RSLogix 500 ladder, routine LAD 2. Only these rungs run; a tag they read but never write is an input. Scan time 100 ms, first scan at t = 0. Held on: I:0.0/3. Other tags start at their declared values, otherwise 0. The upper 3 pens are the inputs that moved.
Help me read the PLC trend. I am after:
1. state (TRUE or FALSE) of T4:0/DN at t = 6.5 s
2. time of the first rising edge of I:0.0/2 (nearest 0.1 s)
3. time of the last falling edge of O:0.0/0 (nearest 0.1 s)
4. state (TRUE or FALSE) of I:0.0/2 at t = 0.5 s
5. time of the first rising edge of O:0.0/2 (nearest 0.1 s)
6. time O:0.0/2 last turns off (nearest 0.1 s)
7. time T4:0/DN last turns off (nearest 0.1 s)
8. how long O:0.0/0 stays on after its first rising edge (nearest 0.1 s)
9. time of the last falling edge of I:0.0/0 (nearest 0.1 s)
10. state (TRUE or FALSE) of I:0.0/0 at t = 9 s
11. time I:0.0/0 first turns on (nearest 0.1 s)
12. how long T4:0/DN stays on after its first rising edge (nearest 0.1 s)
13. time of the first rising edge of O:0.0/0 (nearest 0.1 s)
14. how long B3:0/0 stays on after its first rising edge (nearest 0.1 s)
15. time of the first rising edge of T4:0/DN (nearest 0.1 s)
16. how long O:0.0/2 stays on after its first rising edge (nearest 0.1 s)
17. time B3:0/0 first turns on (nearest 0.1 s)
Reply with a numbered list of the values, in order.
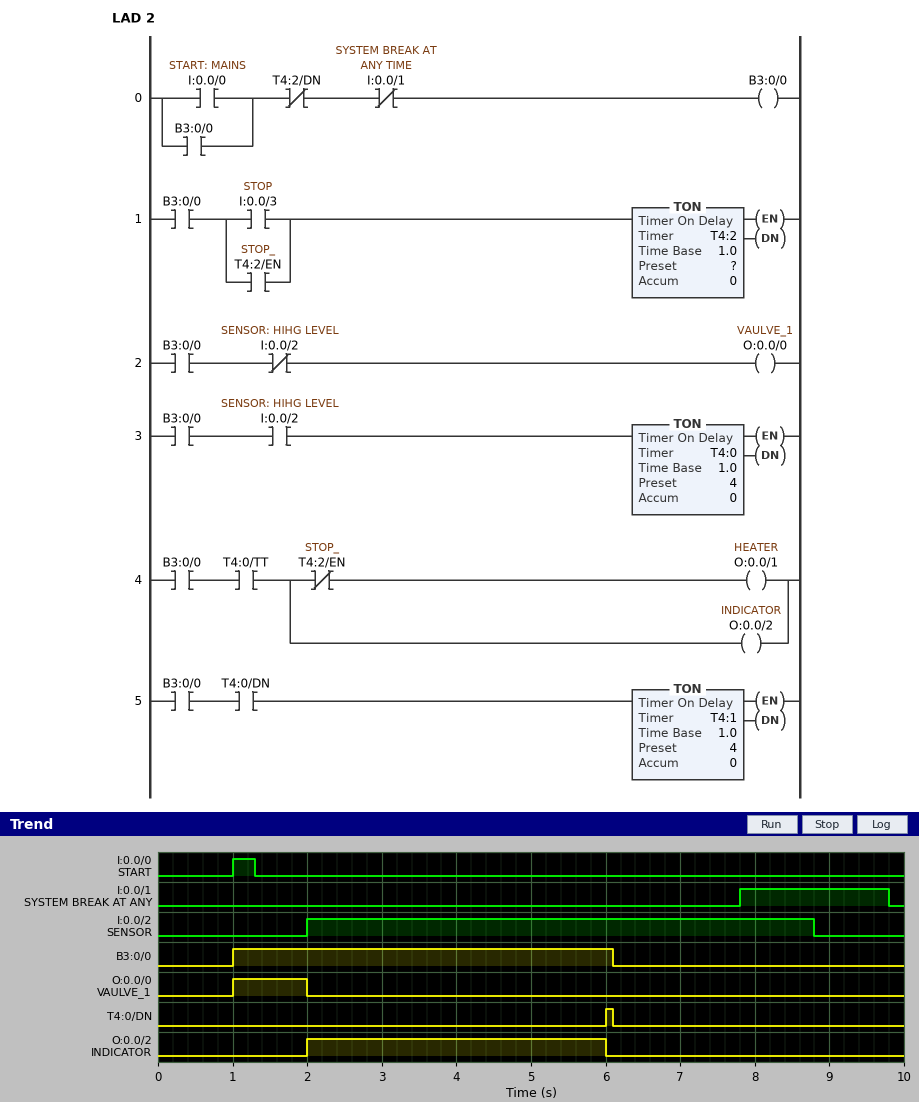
1. FALSE
2. 2.0 s
3. 2.0 s
4. FALSE
5. 2.0 s
6. 6.0 s
7. 6.1 s
8. 1.0 s
9. 1.3 s
10. FALSE
11. 1.0 s
12. 0.1 s
13. 1.0 s
14. 5.1 s
15. 6.0 s
16. 4.0 s
17. 1.0 s
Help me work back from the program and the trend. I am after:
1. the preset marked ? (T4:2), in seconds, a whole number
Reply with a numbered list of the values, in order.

1. 5 s
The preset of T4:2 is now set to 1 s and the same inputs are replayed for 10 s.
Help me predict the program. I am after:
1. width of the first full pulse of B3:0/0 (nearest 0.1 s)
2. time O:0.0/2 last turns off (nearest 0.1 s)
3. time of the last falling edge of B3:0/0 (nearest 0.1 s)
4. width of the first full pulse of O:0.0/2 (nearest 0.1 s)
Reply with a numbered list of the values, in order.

1. 1.1 s
2. 2.1 s
3. 2.1 s
4. 0.1 s
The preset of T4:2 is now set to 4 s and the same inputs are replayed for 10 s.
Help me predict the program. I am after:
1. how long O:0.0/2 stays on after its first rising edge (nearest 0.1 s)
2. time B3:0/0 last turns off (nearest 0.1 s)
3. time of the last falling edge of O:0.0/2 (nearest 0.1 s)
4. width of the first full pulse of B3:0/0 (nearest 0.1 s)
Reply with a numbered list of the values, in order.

1. 3.1 s
2. 5.1 s
3. 5.1 s
4. 4.1 s
